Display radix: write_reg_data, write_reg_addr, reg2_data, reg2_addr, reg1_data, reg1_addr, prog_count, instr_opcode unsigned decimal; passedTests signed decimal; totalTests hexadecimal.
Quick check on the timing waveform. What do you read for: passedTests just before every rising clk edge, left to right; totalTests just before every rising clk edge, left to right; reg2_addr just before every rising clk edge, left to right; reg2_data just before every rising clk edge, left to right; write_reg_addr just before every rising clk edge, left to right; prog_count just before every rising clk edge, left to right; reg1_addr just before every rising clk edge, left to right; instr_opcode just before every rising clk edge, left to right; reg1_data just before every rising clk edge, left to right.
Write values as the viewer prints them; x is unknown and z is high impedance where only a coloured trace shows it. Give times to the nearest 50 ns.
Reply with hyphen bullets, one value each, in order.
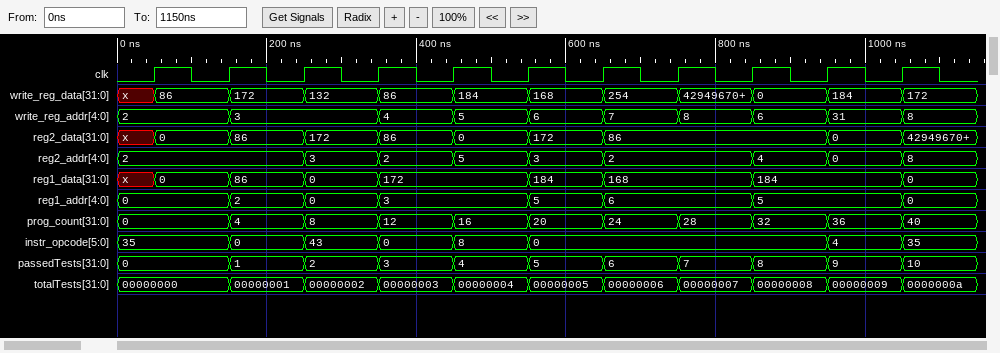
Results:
- 0, 0, 1, 2, 3, 4, 5, 6, 7, 8, 9
- 00000000, 00000000, 00000001, 00000002, 00000003, 00000004, 00000005, 00000006, 00000007, 00000008, 00000009
- 2, 2, 2, 3, 2, 5, 3, 2, 2, 4, 0
- x, 0, 86, 172, 86, 0, 172, 86, 86, 86, 0
- 2, 2, 3, 3, 4, 5, 6, 7, 8, 6, 31
- 0, 0, 4, 8, 12, 16, 20, 24, 28, 32, 36
- 0, 0, 2, 0, 3, 3, 5, 6, 6, 5, 5
- 35, 35, 0, 43, 0, 8, 0, 0, 0, 0, 4
- x, 0, 86, 0, 172, 172, 184, 168, 168, 184, 184
